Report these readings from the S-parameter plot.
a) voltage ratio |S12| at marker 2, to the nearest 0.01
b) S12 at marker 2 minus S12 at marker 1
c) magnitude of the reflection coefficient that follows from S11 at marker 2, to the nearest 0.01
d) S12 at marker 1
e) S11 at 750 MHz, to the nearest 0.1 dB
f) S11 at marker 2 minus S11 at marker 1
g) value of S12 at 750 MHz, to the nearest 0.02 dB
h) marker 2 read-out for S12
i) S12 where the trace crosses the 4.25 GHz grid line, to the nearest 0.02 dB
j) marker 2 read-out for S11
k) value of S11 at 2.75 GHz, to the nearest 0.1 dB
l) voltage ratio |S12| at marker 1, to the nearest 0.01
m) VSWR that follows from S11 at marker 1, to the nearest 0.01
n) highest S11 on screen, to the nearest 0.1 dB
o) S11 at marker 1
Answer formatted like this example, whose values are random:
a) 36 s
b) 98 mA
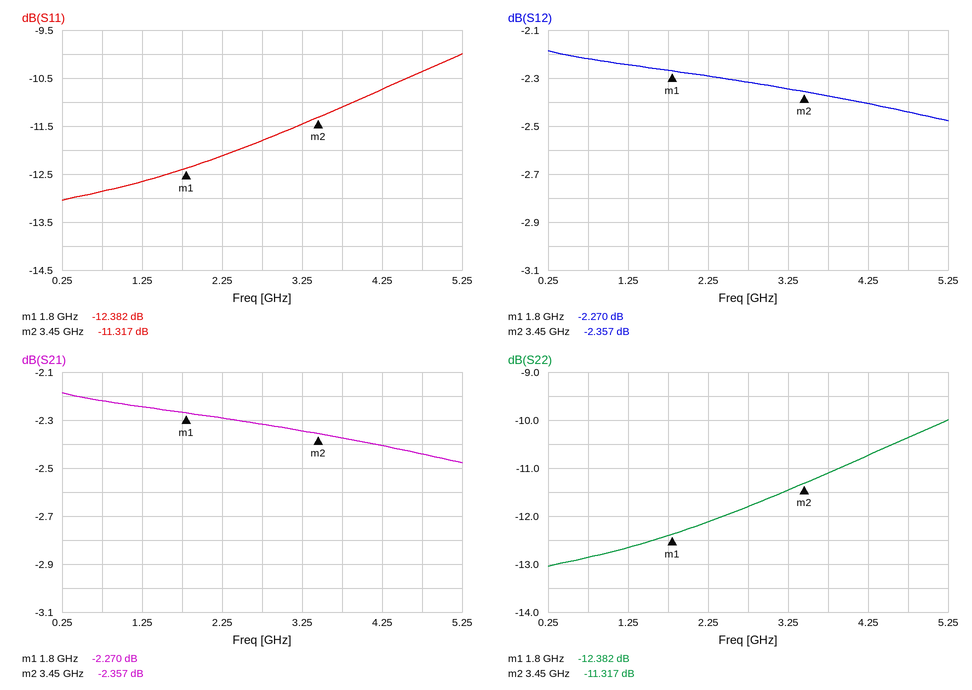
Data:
a) 0.76
b) -0.087 dB
c) 0.27
d) -2.270 dB
e) -12.9 dB
f) 1.065 dB
g) -2.22 dB
h) -2.357 dB
i) -2.40 dB
j) -11.317 dB
k) -11.8 dB
l) 0.77
m) 1.63
n) -10.0 dB
o) -12.382 dB
